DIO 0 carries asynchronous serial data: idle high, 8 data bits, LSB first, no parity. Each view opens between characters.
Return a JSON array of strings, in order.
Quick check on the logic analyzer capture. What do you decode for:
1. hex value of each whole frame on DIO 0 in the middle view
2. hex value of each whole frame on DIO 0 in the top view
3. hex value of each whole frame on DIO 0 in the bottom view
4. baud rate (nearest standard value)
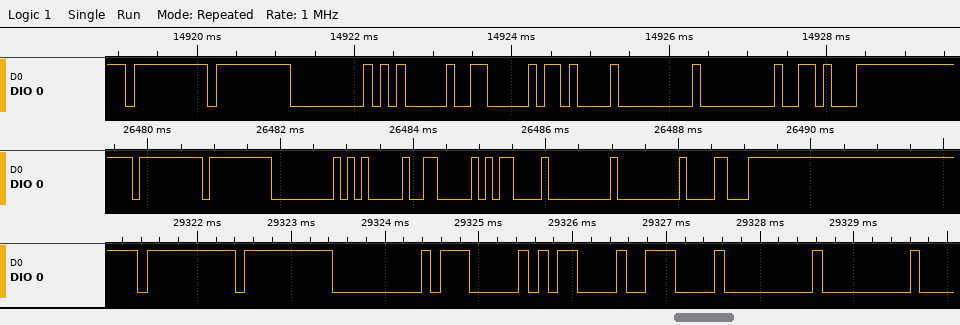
["FF, FF, 00, 05, 06, 0D, 00, 00, 18", "FF, FF, 00, 05, 06, 0B, 00, 00, 16", "FF, FF, 00, 07, 0D, 0E, 00, 00", "9600 baud"]
